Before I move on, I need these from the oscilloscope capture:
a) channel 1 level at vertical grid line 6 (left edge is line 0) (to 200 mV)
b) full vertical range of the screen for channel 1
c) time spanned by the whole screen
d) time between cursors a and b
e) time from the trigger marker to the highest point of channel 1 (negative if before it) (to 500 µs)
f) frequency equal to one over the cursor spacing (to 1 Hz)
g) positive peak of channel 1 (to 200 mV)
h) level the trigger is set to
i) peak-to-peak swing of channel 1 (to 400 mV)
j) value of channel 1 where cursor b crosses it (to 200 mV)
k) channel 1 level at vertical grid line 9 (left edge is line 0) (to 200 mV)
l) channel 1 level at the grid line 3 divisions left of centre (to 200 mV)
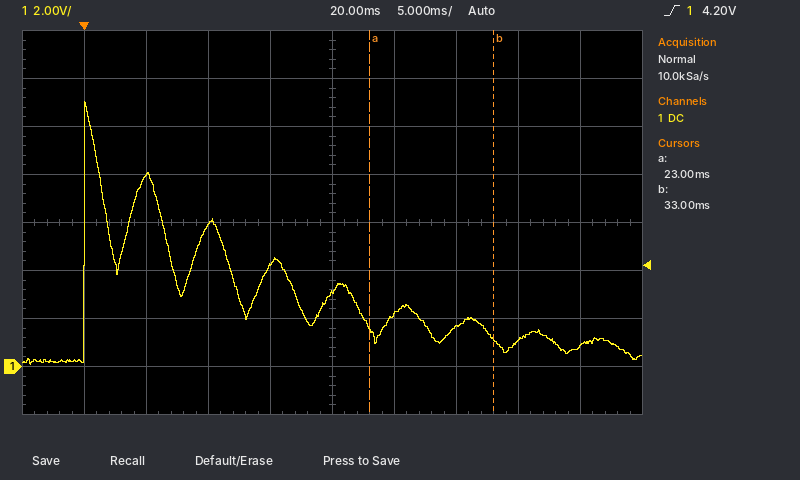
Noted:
2.2 V
16 V
50 ms
10.0 ms
0.0 ms
100 Hz
11.0 V
4.20 V
10.8 V
1.2 V
800 mV
8.0 V
